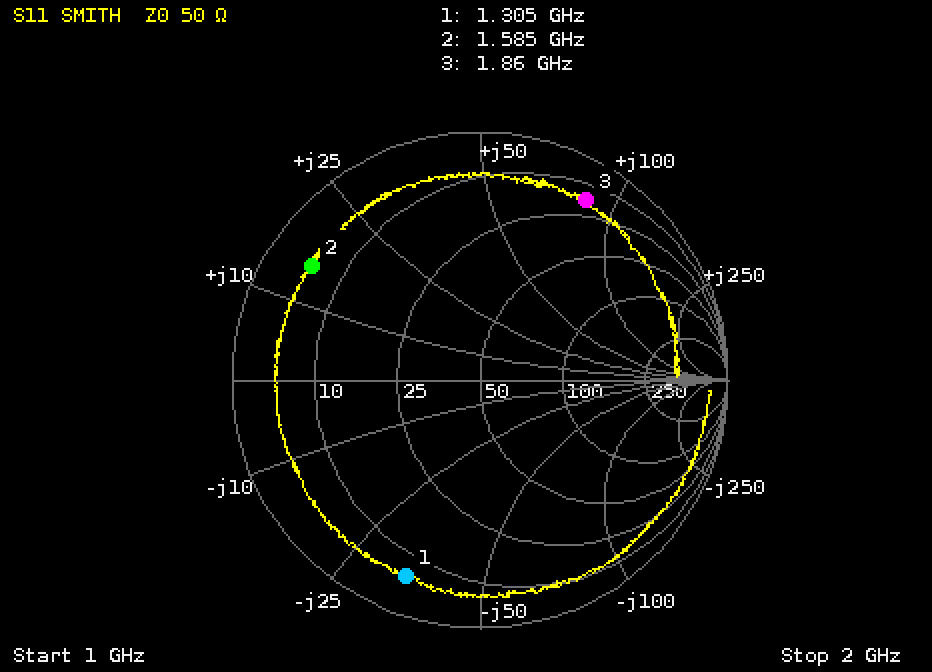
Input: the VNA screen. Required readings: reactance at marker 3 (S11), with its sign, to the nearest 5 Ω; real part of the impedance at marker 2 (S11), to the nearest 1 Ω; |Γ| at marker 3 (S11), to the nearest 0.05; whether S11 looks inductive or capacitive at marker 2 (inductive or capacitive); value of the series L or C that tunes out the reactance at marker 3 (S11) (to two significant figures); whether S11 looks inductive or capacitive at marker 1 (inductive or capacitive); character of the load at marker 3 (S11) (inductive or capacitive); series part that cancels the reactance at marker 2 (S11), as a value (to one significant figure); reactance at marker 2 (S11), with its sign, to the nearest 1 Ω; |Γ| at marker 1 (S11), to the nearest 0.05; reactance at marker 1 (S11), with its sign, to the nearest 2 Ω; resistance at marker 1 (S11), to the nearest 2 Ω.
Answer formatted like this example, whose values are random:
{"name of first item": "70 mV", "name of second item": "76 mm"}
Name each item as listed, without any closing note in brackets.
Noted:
{"reactance at marker 3 (S11), with its sign, to the nearest 5 Ω": "+85 Ω", "real part of the impedance at marker 2 (S11), to the nearest 1 Ω": "5 Ω", "|Γ| at marker 3 (S11), to the nearest 0.05": "0.85", "whether S11 looks inductive or capacitive at marker 2": "inductive", "value of the series L or C that tunes out the reactance at marker 3 (S11)": "1.0 pF", "whether S11 looks inductive or capacitive at marker 1": "capacitive", "character of the load at marker 3 (S11)": "inductive", "series part that cancels the reactance at marker 2 (S11), as a value": "7 pF", "reactance at marker 2 (S11), with its sign, to the nearest 1 Ω": "+15 Ω", "|Γ| at marker 1 (S11), to the nearest 0.05": "0.85", "reactance at marker 1 (S11), with its sign, to the nearest 2 Ω": "-34 Ω", "resistance at marker 1 (S11), to the nearest 2 Ω": "6 Ω"}
